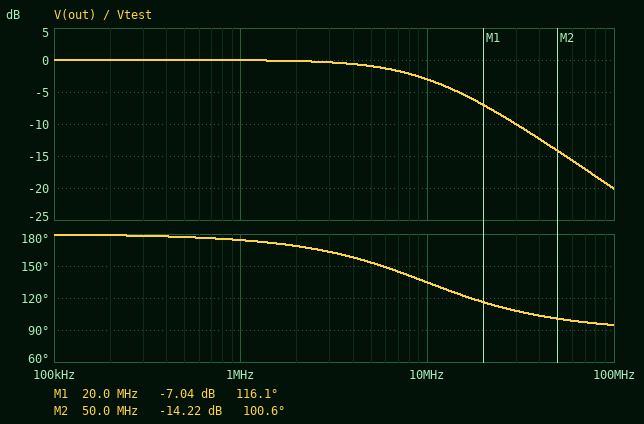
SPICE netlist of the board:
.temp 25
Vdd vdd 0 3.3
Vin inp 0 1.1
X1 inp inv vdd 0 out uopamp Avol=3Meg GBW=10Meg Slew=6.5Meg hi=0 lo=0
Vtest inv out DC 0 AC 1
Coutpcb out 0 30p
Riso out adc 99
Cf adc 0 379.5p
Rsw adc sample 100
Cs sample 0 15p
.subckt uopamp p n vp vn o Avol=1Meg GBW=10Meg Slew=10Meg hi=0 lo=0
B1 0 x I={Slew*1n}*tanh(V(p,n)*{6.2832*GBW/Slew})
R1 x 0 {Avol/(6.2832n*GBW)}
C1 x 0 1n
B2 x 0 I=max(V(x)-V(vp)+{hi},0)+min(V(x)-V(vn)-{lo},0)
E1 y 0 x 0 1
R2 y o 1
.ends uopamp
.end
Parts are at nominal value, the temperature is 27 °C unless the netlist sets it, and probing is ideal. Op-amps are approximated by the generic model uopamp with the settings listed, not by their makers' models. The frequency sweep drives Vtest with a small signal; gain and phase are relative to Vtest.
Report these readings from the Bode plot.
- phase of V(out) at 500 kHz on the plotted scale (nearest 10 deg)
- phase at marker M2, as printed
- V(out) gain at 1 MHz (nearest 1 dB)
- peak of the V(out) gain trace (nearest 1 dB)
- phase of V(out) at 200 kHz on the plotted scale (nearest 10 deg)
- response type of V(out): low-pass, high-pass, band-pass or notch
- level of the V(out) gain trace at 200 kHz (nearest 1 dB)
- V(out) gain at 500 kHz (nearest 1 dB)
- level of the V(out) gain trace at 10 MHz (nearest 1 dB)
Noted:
180 deg
100.6 deg
0 dB
0 dB
180 deg
low-pass
0 dB
0 dB
-3 dB
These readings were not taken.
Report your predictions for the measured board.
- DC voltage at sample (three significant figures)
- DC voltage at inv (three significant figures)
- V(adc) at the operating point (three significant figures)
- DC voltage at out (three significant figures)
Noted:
1.10 V
1.10 V
1.10 V
1.10 V
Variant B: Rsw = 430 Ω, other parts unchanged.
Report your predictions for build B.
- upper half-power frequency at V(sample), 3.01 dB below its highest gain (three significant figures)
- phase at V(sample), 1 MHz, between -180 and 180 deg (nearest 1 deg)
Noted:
3.51 MHz
158 deg
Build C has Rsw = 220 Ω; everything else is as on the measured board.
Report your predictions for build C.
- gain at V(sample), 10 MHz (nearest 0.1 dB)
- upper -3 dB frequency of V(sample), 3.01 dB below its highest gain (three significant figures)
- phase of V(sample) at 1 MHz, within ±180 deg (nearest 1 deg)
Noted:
-11.7 dB
3.56 MHz
159 deg
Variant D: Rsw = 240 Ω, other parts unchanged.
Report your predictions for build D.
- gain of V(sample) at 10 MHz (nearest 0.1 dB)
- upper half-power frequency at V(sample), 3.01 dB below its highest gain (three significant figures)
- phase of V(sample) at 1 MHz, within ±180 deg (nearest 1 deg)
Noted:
-11.7 dB
3.56 MHz
159 deg
